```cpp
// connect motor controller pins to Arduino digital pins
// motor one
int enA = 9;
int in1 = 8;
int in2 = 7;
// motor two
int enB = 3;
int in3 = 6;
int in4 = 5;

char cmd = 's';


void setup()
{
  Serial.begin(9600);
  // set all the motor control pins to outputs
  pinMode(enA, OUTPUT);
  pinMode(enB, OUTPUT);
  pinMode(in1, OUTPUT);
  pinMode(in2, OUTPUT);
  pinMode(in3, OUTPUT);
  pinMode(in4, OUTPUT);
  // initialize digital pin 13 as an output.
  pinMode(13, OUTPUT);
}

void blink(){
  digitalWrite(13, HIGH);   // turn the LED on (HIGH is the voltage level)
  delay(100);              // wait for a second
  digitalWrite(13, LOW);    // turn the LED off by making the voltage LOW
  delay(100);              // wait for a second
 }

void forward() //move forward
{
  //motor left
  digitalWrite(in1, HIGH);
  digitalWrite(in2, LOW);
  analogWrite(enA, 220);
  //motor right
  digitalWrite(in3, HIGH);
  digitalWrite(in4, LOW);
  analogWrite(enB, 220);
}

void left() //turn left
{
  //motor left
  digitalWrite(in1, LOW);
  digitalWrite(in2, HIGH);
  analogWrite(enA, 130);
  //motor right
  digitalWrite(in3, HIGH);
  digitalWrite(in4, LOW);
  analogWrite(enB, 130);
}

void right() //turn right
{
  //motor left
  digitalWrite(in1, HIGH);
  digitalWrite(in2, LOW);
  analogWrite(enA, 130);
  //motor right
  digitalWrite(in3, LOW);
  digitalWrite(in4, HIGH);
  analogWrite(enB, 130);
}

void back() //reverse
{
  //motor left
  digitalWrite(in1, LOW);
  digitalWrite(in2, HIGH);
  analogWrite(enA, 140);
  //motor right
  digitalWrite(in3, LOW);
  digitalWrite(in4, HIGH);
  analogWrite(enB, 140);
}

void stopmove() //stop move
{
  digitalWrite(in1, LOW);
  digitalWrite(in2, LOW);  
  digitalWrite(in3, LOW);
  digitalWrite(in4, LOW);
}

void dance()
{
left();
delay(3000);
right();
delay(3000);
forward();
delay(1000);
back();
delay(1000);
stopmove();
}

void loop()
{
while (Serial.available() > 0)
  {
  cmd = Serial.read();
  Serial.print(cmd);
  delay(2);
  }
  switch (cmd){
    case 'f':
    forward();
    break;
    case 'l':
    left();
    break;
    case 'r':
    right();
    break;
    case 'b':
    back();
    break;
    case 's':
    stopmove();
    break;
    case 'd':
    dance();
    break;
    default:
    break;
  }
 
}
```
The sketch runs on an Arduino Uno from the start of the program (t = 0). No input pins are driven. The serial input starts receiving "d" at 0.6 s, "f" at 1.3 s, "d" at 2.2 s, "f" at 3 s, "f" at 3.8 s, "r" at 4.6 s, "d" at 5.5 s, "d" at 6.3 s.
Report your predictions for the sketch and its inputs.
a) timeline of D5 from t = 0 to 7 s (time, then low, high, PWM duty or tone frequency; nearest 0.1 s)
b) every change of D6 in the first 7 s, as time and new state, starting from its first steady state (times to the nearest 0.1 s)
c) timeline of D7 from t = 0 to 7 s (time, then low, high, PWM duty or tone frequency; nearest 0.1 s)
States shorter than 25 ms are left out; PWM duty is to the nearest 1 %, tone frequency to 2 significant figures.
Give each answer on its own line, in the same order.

0 s low; 3.6 s high; 6.6 s low
0 s low; 0.6 s high; 3.6 s low; 6.6 s high
0 s low; 0.6 s high; 3.6 s low
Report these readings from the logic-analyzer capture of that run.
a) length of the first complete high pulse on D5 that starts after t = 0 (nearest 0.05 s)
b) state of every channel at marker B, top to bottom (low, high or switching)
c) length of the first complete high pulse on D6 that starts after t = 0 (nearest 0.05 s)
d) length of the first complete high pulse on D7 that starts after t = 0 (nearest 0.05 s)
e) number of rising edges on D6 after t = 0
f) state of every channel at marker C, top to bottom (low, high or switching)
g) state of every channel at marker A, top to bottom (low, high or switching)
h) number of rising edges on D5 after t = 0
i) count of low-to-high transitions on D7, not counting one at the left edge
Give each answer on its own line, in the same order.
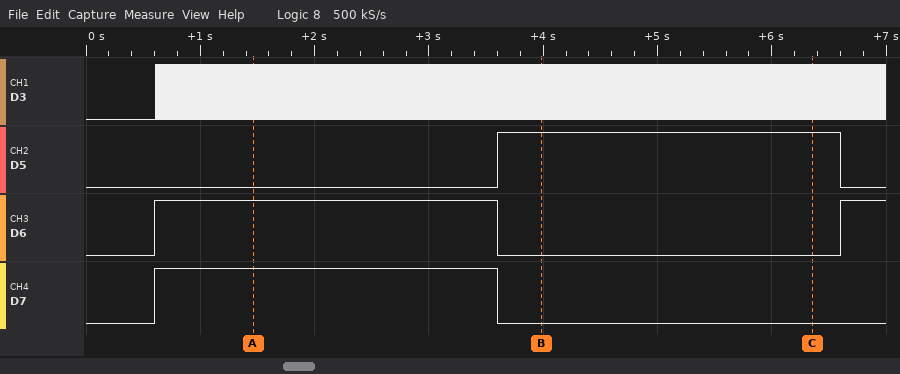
3.00 s
D3 switching, D5 high, D6 low, D7 low
3.00 s
3.00 s
2
D3 switching, D5 high, D6 low, D7 low
D3 switching, D5 low, D6 high, D7 high
1
1
